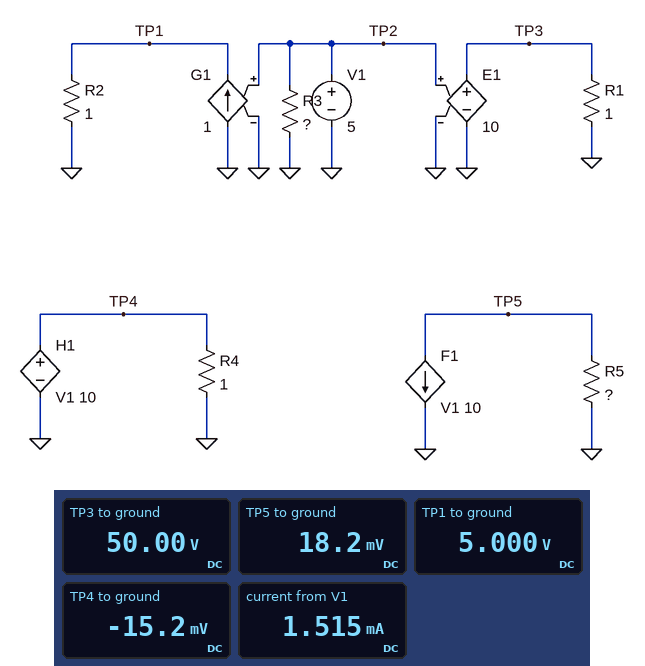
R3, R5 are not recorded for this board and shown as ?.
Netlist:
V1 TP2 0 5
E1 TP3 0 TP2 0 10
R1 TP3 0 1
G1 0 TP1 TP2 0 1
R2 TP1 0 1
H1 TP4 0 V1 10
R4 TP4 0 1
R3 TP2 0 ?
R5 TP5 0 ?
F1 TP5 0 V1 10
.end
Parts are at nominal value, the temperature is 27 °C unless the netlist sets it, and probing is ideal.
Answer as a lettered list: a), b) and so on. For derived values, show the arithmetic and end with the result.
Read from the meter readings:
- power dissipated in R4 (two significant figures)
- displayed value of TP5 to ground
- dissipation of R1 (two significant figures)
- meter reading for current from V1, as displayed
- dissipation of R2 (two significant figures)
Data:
a) (0 V - (-15.2 mV))^2 / 1 Ω = 230 µW
b) 18.2 mV
c) (50 V)^2 / 1 Ω = 2.5 kW
d) 1.515 mA
e) (5 V)^2 / 1 Ω = 25 W
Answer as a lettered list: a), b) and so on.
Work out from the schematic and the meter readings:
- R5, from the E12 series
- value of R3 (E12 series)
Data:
a) 1.2 Ω
b) 3.3 kΩ
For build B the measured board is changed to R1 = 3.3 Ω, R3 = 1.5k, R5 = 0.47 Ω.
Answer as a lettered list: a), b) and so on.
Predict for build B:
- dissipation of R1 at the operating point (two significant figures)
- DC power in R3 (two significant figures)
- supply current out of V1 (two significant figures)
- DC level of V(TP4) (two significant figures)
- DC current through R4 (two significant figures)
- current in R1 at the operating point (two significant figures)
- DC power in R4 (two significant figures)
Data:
a) 760 W
b) 17 mW
c) 3.3 mA
d) -33 mV
e) 33 mA
f) 15 A
g) 1.1 mW
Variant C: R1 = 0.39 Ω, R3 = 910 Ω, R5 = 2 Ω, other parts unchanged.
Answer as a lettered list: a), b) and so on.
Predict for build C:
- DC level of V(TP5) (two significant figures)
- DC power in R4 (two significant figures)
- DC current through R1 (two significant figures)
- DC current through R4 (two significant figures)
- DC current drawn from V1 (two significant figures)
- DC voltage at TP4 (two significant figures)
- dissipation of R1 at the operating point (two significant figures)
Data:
a) 110 mV
b) 3.0 mW
c) 130 A
d) 55 mA
e) 5.5 mA
f) -55 mV
g) 6.4 kW
